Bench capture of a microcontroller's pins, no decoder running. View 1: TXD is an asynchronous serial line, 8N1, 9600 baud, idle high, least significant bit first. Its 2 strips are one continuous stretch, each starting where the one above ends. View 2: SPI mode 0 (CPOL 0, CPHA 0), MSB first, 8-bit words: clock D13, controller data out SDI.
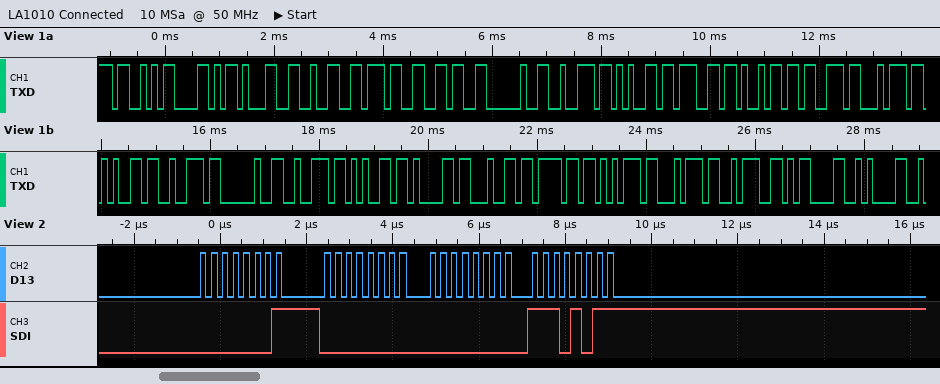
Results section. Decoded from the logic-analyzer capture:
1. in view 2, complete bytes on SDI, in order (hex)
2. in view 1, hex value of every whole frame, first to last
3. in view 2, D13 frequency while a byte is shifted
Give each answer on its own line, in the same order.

01 00 00 EB
53 58 31 32 37 36 20 72 65 67 69 73 74 65 72 20 72 65 61 64 6F 75 74 3A 0D 0A
4 MHz
